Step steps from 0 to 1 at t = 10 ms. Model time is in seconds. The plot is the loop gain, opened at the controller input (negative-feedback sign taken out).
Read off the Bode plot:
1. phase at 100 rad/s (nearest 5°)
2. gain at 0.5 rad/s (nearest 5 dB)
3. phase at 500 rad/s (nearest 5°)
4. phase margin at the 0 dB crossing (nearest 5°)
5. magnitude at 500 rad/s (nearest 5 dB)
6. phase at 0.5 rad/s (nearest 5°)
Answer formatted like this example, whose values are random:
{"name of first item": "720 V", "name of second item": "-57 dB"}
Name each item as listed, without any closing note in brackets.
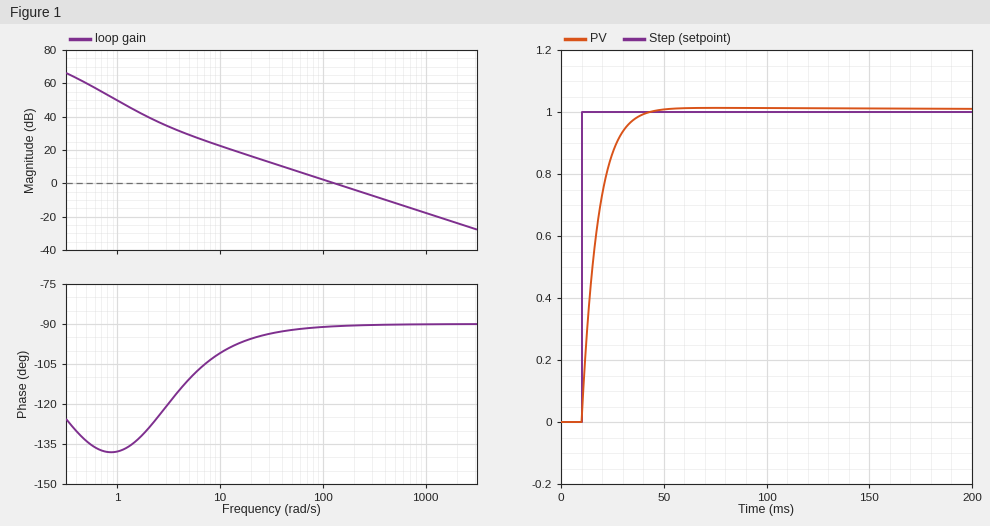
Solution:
{"phase at 100 rad/s": "-90°", "gain at 0.5 rad/s": "60 dB", "phase at 500 rad/s": "-90°", "phase margin at the 0 dB crossing": "90°", "magnitude at 500 rad/s": "-10 dB", "phase at 0.5 rad/s": "-135°"}
